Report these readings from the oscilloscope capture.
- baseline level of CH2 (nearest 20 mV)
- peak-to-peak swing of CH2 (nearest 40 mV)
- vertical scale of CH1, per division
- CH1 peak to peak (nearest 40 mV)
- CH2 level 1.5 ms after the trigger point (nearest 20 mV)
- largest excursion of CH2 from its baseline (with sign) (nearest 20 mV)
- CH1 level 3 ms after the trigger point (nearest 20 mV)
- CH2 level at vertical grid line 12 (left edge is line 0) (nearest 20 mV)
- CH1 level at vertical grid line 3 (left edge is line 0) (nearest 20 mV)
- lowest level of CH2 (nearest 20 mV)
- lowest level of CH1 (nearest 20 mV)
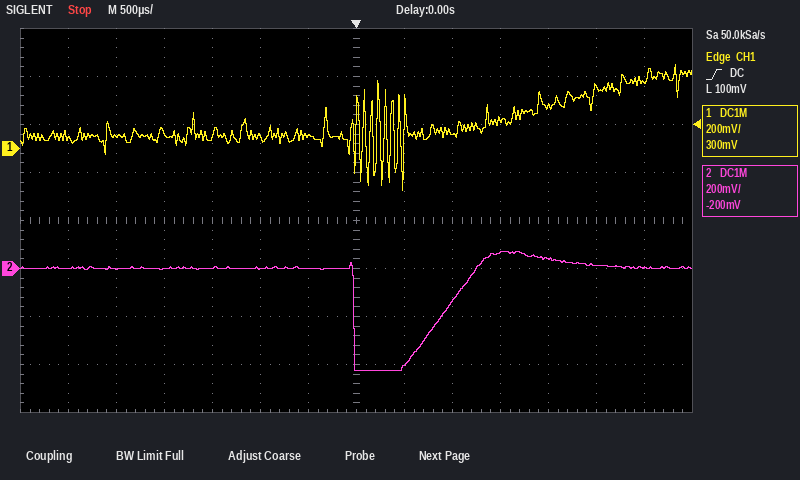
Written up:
0 mV
480 mV
200 mV
520 mV
60 mV
-420 mV
280 mV
20 mV
60 mV
-420 mV
-180 mV
